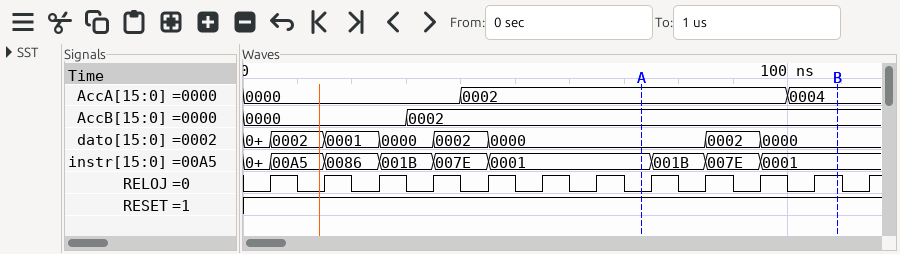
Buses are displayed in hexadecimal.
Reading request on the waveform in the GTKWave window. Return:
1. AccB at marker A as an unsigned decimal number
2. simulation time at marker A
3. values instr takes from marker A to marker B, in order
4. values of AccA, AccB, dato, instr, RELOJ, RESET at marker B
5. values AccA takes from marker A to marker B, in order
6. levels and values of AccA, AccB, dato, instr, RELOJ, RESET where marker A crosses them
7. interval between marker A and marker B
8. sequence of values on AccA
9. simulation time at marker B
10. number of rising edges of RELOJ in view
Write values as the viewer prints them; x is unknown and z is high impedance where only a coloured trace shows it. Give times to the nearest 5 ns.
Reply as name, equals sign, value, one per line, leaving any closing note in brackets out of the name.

AccB at marker A as an unsigned decimal number = 2
simulation time at marker A = 75 ns
values instr takes from marker A to marker B, in order = 0001, 001B, 007E, 0001
values of AccA, AccB, dato, instr, RELOJ, RESET at marker B = AccA=0004, AccB=0002, dato=0000, instr=0001, RELOJ=1, RESET=1
values AccA takes from marker A to marker B, in order = 0002, 0004
levels and values of AccA, AccB, dato, instr, RELOJ, RESET where marker A crosses them = AccA=0002, AccB=0002, dato=0000, instr=0001, RELOJ=0, RESET=1
interval between marker A and marker B = 35 ns
sequence of values on AccA = 0000, 0002, 0004
simulation time at marker B = 110 ns
number of rising edges of RELOJ in view = 12
